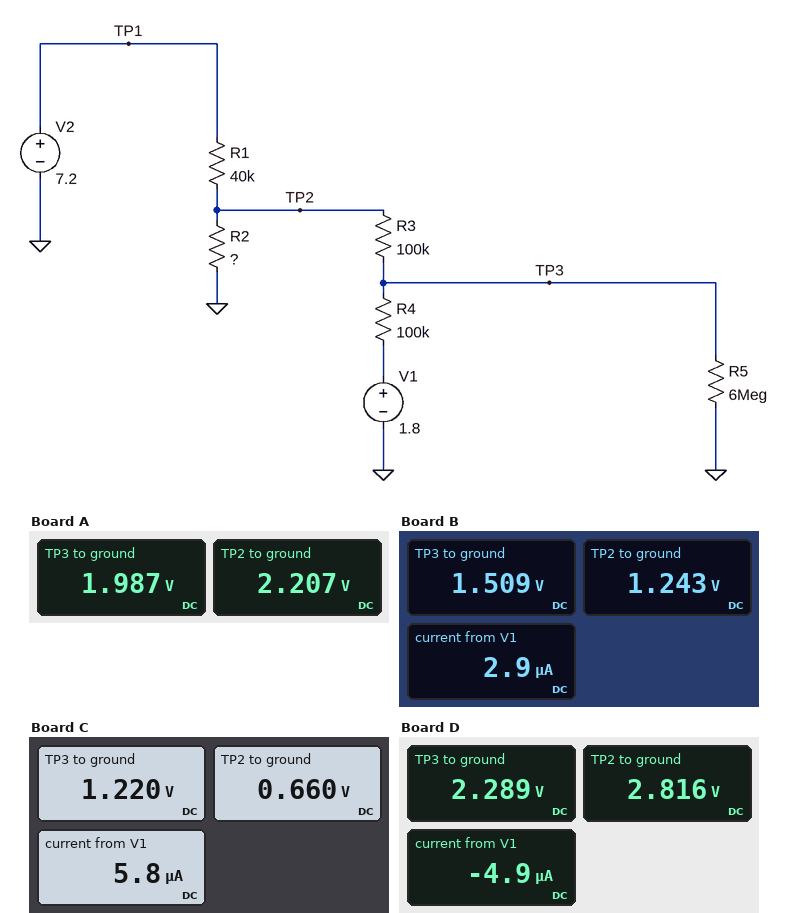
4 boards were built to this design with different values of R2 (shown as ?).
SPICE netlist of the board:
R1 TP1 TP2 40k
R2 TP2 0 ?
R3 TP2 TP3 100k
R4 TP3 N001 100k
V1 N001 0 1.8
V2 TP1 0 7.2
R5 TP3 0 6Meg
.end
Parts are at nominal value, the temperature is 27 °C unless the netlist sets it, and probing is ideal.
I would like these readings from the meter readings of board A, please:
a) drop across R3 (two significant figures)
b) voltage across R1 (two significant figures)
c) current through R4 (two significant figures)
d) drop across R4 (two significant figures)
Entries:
220 mV
5.0 V
1.9 µA
190 mV
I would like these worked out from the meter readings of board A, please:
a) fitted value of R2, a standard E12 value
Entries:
18 kΩ
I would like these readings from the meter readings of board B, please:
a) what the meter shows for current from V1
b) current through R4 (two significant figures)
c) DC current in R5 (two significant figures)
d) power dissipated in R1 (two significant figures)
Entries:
2.9 µA
2.9 µA
250 nA
890 µW
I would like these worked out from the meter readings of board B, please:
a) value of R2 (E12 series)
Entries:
8.2 kΩ
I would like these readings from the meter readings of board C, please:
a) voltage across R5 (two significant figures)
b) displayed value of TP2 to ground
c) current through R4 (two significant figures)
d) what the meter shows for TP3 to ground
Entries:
1.2 V
0.660 V
5.8 µA
1.220 V
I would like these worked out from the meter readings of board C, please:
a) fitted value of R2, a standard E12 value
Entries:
3.9 kΩ
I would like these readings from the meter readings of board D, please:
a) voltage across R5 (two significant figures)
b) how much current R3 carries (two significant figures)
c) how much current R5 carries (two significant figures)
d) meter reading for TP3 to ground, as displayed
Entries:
2.3 V
5.3 µA
380 nA
2.289 V
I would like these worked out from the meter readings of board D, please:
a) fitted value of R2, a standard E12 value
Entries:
27 kΩ
